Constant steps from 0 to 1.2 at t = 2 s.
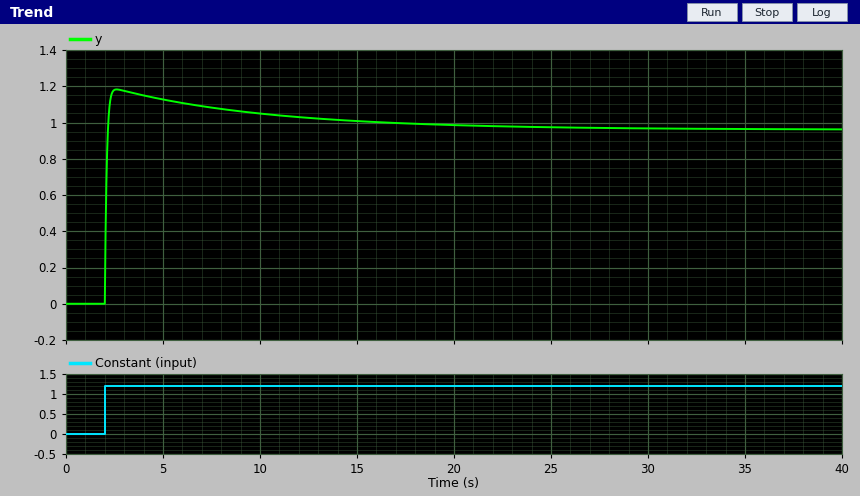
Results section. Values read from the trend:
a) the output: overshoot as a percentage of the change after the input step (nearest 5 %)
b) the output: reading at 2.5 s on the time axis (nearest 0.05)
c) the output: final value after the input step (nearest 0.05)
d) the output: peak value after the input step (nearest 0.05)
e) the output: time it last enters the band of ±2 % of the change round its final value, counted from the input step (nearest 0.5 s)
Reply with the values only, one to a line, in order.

25 %
1.20
0.95
1.20
20.5 s
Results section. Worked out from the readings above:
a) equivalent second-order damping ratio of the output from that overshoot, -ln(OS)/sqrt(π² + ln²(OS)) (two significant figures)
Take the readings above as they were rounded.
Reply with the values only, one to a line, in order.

0.40
